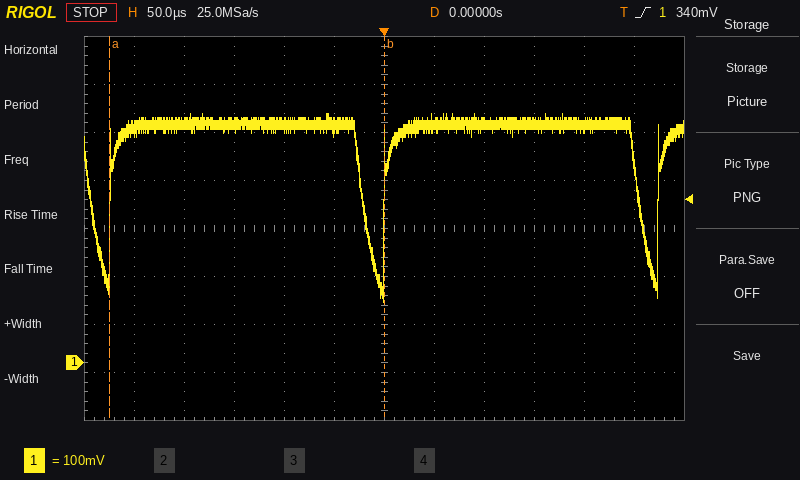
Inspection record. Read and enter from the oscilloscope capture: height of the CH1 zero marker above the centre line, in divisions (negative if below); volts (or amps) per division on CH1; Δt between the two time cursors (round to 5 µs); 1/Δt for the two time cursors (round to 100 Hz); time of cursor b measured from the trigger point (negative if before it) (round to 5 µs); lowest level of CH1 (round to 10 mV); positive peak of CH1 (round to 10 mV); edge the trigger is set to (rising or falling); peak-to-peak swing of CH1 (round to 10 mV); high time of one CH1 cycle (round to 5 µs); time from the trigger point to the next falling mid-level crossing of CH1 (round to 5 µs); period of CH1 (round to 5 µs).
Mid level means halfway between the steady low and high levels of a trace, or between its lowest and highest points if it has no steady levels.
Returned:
-2.8 div
100 mV
275 µs
3.6 kHz
0 µs
130 mV
520 mV
rising
390 mV
255 µs
255 µs
275 µs
